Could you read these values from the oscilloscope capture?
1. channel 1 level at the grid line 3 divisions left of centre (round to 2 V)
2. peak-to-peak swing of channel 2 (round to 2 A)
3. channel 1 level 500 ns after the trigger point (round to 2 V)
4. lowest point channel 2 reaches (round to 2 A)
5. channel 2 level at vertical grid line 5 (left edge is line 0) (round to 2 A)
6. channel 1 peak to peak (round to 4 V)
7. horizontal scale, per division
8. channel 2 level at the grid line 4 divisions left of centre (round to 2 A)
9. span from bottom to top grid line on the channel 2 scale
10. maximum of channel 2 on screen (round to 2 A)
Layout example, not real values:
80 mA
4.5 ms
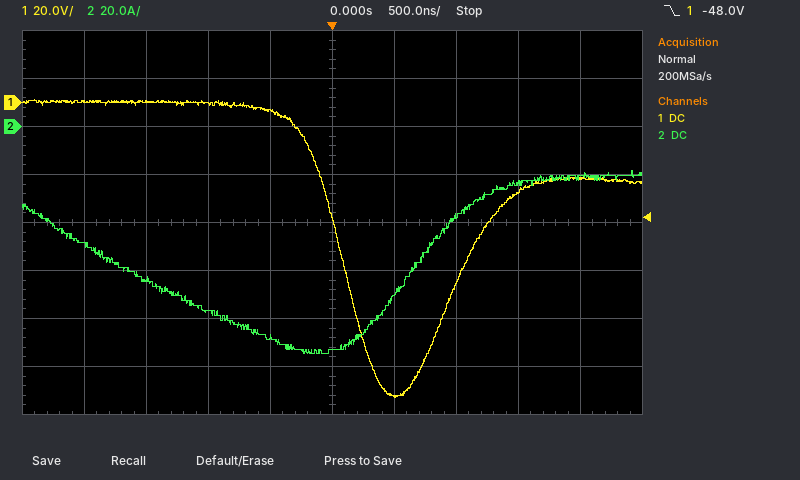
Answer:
0 V
76 A
-122 V
-94 A
-92 A
124 V
500 ns
-50 A
160 A
-18 A
